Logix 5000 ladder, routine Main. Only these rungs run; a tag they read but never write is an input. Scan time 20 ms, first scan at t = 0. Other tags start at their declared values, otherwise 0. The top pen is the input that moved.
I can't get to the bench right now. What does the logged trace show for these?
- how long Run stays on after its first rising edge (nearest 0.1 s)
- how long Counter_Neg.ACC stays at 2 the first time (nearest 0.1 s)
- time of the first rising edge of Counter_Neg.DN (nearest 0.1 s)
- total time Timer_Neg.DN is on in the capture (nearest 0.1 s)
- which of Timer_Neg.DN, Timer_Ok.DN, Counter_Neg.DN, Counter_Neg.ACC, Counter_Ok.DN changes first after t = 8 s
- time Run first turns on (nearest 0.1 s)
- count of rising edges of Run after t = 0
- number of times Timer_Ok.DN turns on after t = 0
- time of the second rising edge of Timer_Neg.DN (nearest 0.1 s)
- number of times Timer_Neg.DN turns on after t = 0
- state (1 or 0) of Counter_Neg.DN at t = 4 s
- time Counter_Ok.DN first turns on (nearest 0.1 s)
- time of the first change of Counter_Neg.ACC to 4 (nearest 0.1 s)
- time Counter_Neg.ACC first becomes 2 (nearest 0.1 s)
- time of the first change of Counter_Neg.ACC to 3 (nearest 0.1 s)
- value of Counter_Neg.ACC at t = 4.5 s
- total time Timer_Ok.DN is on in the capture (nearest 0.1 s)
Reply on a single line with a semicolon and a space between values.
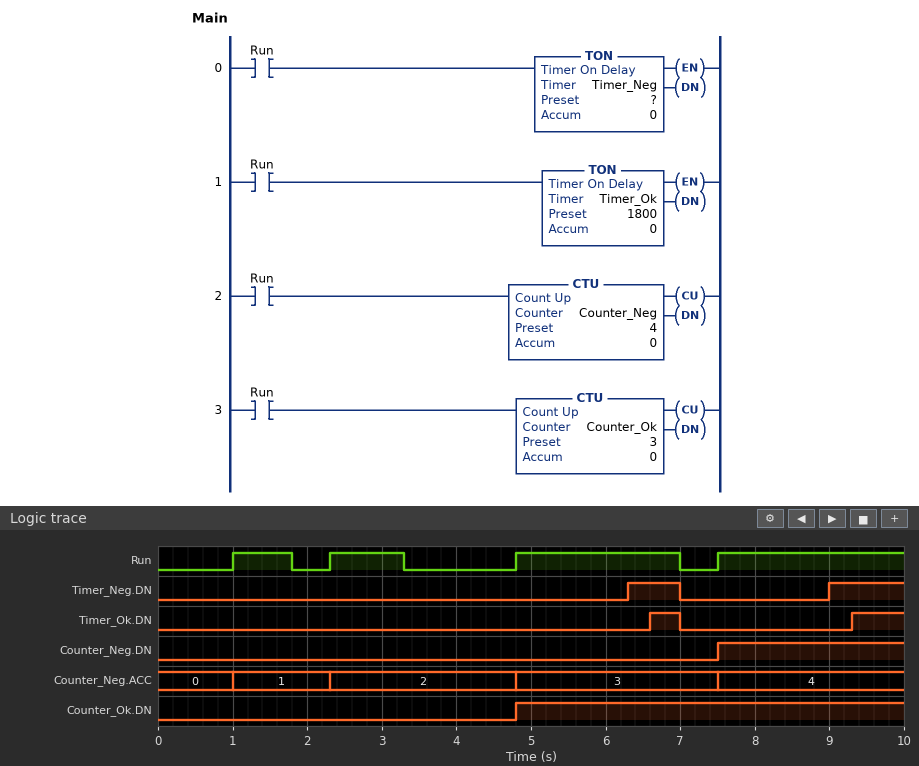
0.8 s; 2.5 s; 7.5 s; 1.7 s; Timer_Neg.DN; 1.0 s; 4; 2; 9.0 s; 2; 0; 4.8 s; 7.5 s; 2.3 s; 4.8 s; 2; 1.1 s
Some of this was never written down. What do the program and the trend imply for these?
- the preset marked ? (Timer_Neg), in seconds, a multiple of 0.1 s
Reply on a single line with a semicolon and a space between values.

1.5 s
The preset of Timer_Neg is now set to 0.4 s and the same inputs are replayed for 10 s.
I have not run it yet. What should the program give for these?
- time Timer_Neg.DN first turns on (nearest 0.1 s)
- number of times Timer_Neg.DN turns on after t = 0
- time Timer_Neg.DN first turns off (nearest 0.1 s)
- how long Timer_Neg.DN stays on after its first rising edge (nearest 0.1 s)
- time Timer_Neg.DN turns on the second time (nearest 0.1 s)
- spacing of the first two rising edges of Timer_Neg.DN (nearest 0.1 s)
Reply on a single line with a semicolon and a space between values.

1.4 s; 4; 1.8 s; 0.4 s; 2.7 s; 1.3 s
